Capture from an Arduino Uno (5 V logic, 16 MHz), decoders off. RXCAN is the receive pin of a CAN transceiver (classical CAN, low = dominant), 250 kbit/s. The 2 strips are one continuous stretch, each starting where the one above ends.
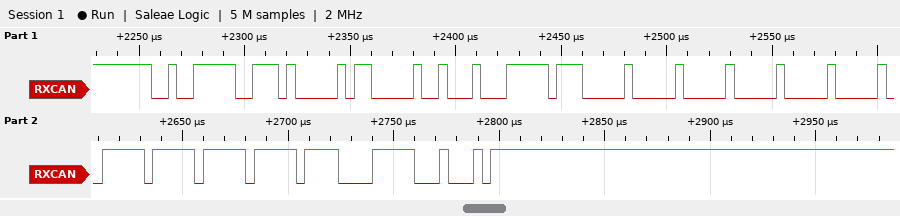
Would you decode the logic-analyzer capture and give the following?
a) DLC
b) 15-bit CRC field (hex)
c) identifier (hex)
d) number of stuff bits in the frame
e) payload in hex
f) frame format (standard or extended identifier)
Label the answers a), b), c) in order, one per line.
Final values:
a) 8
b) 0x07C8
c) 0x09F50301
d) 15
e) FF 00 00 00 00 FF FF FF
f) extended
